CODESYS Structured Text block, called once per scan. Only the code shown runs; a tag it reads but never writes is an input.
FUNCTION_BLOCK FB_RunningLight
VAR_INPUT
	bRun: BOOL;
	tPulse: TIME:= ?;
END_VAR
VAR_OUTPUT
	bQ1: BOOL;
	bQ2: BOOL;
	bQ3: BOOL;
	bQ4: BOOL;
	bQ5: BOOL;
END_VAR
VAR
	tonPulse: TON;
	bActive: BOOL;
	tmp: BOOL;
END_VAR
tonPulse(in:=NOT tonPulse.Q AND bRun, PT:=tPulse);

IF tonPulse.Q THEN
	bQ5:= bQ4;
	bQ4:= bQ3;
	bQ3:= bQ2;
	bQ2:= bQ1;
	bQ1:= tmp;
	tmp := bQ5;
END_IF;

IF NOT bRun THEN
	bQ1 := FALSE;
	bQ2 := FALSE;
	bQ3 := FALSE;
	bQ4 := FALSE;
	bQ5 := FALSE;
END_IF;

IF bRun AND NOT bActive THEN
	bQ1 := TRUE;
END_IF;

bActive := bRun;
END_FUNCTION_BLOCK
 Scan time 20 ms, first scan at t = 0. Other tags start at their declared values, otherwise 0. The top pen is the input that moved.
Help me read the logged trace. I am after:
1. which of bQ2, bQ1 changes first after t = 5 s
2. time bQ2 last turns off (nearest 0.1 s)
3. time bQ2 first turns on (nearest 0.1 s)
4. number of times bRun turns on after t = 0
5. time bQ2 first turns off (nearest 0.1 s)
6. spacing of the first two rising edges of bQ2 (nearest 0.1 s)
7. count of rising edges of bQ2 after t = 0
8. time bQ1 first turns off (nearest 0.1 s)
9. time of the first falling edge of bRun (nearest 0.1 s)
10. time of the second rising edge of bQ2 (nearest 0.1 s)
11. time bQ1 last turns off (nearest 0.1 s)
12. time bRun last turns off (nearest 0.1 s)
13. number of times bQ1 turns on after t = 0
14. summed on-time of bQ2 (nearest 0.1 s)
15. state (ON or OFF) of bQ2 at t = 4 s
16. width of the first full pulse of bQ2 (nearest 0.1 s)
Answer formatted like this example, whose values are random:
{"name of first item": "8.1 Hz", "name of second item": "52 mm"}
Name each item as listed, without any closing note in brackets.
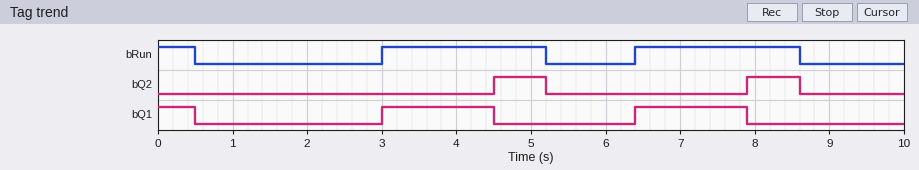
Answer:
{"which of bQ2, bQ1 changes first after t = 5 s": "bQ2", "time bQ2 last turns off": "8.6 s", "time bQ2 first turns on": "4.5 s", "number of times bRun turns on after t = 0": "2", "time bQ2 first turns off": "5.2 s", "spacing of the first two rising edges of bQ2": "3.4 s", "count of rising edges of bQ2 after t = 0": "2", "time bQ1 first turns off": "0.5 s", "time of the first falling edge of bRun": "0.5 s", "time of the second rising edge of bQ2": "7.9 s", "time bQ1 last turns off": "7.9 s", "time bRun last turns off": "8.6 s", "number of times bQ1 turns on after t = 0": "2", "summed on-time of bQ2": "1.4 s", "state (ON or OFF) of bQ2 at t = 4 s": "OFF", "width of the first full pulse of bQ2": "0.7 s"}
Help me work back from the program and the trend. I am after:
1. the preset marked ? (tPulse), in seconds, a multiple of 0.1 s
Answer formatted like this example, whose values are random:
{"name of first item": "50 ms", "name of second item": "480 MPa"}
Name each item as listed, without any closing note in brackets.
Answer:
{"the preset marked ? (tPulse), in seconds, a multiple of 0.1 s": "1.5 s"}
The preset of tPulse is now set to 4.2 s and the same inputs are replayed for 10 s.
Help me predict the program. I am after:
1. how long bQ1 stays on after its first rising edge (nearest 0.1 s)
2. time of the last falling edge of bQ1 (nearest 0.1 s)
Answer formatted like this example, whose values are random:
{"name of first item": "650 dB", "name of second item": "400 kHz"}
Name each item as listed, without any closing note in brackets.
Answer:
{"how long bQ1 stays on after its first rising edge": "2.2 s", "time of the last falling edge of bQ1": "8.6 s"}
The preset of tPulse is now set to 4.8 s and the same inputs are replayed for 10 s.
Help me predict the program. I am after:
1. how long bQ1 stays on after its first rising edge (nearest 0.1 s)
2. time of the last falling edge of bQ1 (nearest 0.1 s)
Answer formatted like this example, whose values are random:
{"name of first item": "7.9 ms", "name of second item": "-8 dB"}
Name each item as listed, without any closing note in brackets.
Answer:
{"how long bQ1 stays on after its first rising edge": "2.2 s", "time of the last falling edge of bQ1": "8.6 s"}
